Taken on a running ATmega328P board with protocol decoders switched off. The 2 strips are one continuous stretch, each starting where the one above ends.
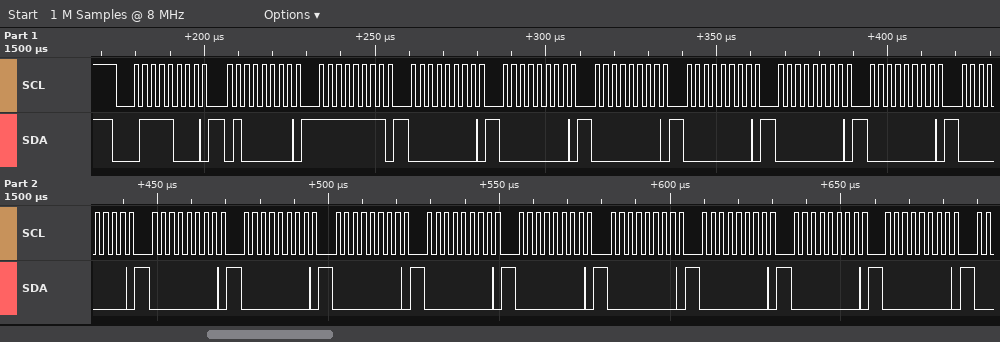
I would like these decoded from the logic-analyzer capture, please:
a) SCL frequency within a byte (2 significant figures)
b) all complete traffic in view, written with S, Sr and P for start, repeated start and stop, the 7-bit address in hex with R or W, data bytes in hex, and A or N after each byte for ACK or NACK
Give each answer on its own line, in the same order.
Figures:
400 kHz
S 3CW A 40 A FF A 00 A 00 A 00 A 00 A 00 A 00 A 00 A 00 A 00 A 00 A 00 A 00 A 00 A 00 A 00 A 00 A
